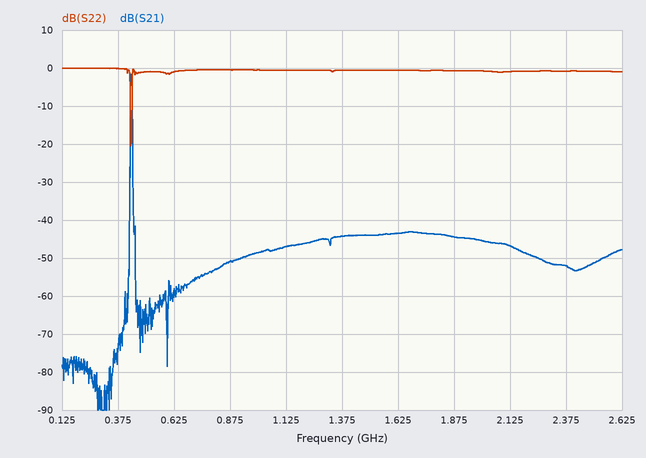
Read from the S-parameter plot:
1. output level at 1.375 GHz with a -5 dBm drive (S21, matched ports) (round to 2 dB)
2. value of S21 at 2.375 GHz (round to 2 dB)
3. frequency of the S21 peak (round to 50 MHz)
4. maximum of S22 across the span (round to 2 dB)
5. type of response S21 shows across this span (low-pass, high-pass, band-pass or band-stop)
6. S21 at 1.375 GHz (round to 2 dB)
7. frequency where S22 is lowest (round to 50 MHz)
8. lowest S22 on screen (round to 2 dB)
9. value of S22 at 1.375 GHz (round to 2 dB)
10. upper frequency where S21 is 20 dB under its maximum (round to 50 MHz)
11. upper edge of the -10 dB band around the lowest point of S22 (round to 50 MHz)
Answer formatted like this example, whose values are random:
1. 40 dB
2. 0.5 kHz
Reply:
1. -50 dBm
2. -52 dB
3. 450 MHz
4. 0 dB
5. band-pass
6. -44 dB
7. 450 MHz
8. -20 dB
9. 0 dB
10. 450 MHz
11. 450 MHz
